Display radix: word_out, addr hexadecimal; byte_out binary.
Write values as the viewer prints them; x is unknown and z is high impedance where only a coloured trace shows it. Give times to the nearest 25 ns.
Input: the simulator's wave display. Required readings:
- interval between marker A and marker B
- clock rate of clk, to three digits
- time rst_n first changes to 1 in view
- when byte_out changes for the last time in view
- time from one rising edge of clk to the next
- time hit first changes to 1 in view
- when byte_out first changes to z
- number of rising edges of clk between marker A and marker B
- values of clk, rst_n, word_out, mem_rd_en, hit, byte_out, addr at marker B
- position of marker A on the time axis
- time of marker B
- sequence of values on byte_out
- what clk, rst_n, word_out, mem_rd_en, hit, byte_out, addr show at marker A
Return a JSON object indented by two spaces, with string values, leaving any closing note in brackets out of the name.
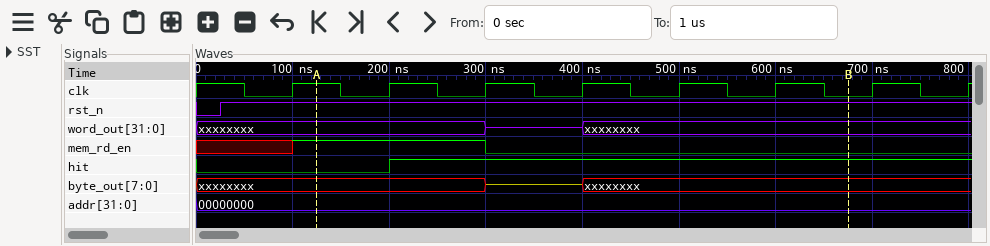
{
  "interval between marker A and marker B": "550 ns",
  "clock rate of clk, to three digits": "10.0 MHz",
  "time rst_n first changes to 1 in view": "25 ns",
  "when byte_out changes for the last time in view": "400 ns",
  "time from one rising edge of clk to the next": "100 ns",
  "time hit first changes to 1 in view": "200 ns",
  "when byte_out first changes to z": "300 ns",
  "number of rising edges of clk between marker A and marker B": "5",
  "values of clk, rst_n, word_out, mem_rd_en, hit, byte_out, addr at marker B": "clk=0, rst_n=1, word_out=xxxxxxxx, mem_rd_en=0, hit=1, byte_out=xxxxxxxx, addr=00000000",
  "position of marker A on the time axis": "125 ns",
  "time of marker B": "675 ns",
  "sequence of values on byte_out": "xxxxxxxx, z, xxxxxxxx",
  "what clk, rst_n, word_out, mem_rd_en, hit, byte_out, addr show at marker A": "clk=1, rst_n=1, word_out=xxxxxxxx, mem_rd_en=1, hit=0, byte_out=xxxxxxxx, addr=00000000"
}
